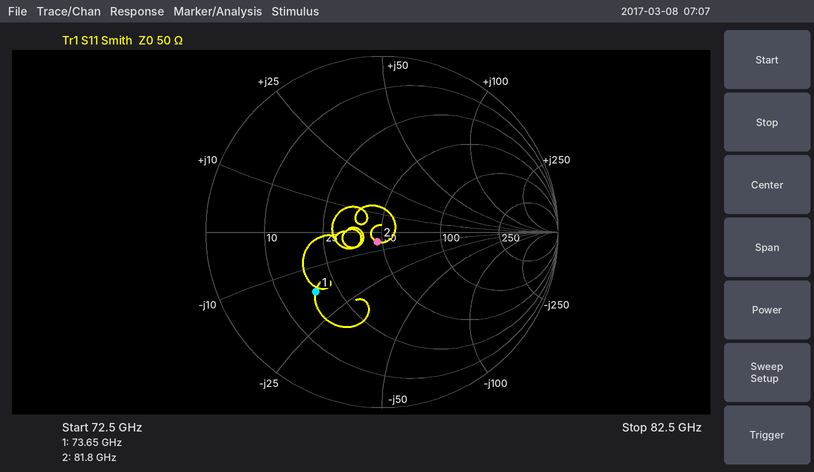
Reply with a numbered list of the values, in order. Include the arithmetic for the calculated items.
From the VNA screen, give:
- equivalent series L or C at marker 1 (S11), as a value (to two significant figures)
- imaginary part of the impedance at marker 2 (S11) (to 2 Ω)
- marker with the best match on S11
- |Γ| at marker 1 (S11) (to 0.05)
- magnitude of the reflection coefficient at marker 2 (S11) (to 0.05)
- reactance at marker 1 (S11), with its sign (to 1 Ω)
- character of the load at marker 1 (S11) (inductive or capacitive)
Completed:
1. C = 1/(2π × 73.65 GHz × 17 Ω) ≈ 127 fF, so 130 fF to two significant figures
2. -6 Ω
3. marker 2
4. 0.50
5. 0.05
6. -17 Ω
7. capacitive
